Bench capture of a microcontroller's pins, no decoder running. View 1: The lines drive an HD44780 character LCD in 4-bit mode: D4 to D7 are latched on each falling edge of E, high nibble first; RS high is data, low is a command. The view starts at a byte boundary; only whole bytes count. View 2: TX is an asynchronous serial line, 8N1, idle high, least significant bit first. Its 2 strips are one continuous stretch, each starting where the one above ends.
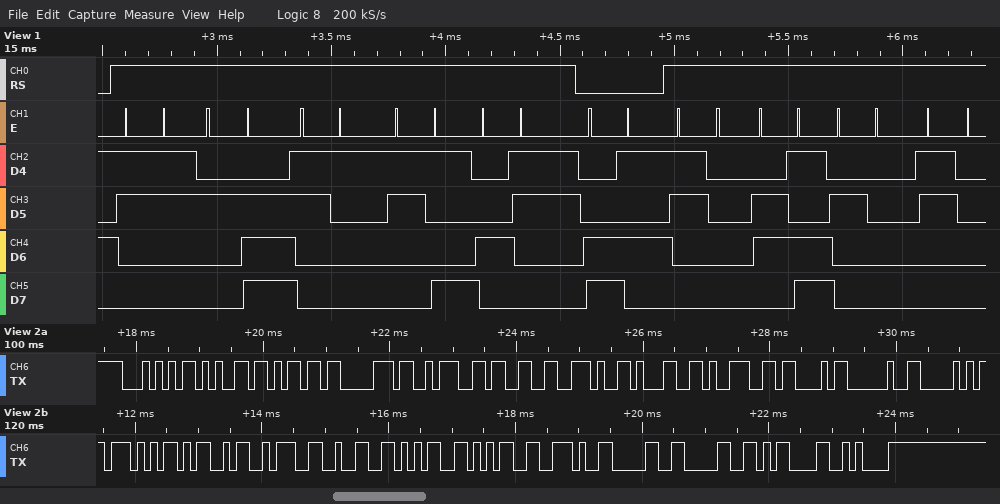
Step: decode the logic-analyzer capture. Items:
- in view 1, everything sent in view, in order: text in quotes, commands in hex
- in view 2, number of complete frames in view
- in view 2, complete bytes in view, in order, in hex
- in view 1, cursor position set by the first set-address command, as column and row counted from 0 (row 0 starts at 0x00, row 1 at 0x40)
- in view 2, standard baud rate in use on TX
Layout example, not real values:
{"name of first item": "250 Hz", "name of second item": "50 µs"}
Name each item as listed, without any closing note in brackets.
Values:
{"in view 1, everything sent in view, in order: text in quotes, commands in hex": "\"3.19C\" 0xC5 \"0m 0\"", "in view 2, number of complete frames in view": "23", "in view 2, complete bytes in view, in order, in hex": "54 65 6D 70 3A 33 2E 31 39 43 20 50 57 4D 3A 32 35 35 2E 30 30 0D 0A", "in view 1, cursor position set by the first set-address command, as column and row counted from 0": "column 5, row 1", "in view 2, standard baud rate in use on TX": "9600 baud"}
